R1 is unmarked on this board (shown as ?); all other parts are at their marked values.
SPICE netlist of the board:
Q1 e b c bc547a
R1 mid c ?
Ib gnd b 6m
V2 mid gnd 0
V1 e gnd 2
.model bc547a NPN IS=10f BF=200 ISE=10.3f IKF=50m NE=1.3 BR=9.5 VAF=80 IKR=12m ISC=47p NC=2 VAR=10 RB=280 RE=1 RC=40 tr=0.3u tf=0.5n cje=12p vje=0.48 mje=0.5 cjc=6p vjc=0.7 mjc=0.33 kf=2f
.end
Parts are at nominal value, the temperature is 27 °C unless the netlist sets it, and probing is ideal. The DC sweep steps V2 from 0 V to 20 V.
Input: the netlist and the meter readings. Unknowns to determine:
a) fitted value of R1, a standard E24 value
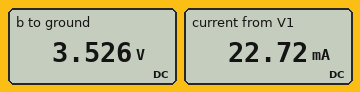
36 Ω
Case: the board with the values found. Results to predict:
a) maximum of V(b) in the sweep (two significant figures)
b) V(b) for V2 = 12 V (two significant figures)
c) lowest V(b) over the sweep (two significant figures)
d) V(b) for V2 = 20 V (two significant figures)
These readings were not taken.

6.6 V
6.0 V
3.5 V
6.6 V
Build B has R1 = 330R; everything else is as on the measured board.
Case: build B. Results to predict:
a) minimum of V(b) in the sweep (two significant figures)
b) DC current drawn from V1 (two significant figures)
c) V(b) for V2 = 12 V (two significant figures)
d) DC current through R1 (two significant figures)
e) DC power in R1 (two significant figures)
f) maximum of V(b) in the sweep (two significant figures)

4.4 V
17 µA
5.6 V
6.0 mA
12 mW
5.9 V
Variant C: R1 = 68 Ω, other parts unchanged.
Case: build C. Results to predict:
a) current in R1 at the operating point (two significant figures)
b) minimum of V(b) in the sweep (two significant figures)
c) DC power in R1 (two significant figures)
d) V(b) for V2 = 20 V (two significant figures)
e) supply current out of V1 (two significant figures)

20 mA
3.9 V
28 mW
6.5 V
14 mA
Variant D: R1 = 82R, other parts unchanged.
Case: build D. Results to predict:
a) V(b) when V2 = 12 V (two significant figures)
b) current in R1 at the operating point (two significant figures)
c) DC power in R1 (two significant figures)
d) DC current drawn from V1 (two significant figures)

5.9 V
18 mA
27 mW
12 mA
